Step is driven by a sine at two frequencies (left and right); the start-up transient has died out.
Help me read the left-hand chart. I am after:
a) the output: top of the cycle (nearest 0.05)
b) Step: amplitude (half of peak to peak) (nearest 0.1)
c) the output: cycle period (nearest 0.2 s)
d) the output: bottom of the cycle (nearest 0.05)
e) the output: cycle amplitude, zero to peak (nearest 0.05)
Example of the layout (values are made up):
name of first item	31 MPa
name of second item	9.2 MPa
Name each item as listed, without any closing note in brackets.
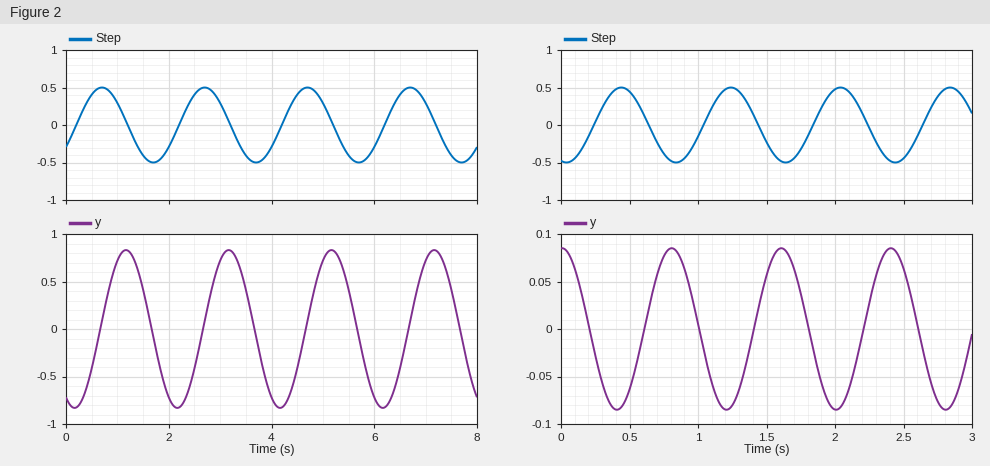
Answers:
the output: top of the cycle	0.85
Step: amplitude (half of peak to peak)	0.5
the output: cycle period	2.0 s
the output: bottom of the cycle	-0.85
the output: cycle amplitude, zero to peak	0.85
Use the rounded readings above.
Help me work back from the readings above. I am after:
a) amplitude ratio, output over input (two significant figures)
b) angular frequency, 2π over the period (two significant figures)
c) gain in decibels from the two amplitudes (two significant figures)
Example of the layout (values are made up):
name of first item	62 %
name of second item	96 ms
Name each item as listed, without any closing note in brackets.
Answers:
amplitude ratio, output over input	1.7
angular frequency, 2π over the period	3.1 rad/s
gain in decibels from the two amplitudes	4.6 dB
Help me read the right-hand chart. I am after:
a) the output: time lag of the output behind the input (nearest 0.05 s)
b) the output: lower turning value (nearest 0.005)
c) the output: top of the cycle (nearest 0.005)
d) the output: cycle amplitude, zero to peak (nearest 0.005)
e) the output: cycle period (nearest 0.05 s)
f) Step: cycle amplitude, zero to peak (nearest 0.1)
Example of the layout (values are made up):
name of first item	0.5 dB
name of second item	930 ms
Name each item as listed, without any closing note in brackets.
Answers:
the output: time lag of the output behind the input	0.35 s
the output: lower turning value	-0.085
the output: top of the cycle	0.085
the output: cycle amplitude, zero to peak	0.085
the output: cycle period	0.80 s
Step: cycle amplitude, zero to peak	0.5
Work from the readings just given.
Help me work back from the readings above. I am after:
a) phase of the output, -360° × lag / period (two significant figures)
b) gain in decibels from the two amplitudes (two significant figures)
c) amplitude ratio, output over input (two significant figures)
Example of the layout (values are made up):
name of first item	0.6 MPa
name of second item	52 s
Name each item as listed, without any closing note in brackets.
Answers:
phase of the output, -360° × lag / period	-160°
gain in decibels from the two amplitudes	-15 dB
amplitude ratio, output over input	0.17
